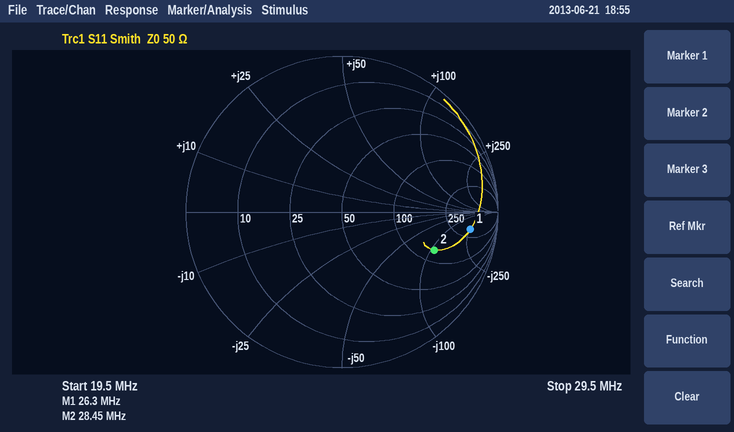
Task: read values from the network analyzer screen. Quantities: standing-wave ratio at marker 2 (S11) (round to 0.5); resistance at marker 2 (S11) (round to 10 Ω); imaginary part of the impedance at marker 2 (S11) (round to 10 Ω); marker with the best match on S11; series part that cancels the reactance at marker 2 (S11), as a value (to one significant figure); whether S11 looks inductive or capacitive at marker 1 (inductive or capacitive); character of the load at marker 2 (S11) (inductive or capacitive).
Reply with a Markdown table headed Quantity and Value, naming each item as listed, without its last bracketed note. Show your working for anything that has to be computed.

| Quantity | Value |
|---|---|
| standing-wave ratio at marker 2 (S11) | 4.5 |
| resistance at marker 2 (S11) | 130 Ω |
| imaginary part of the impedance at marker 2 (S11) | -110 Ω |
| marker with the best match on S11 | marker 2 |
| series part that cancels the reactance at marker 2 (S11), as a value | L = 110 Ω/(2π × 28.45 MHz) ≈ 615 nH, so 600 nH to one significant figure |
| whether S11 looks inductive or capacitive at marker 1 | capacitive |
| character of the load at marker 2 (S11) | capacitive |
